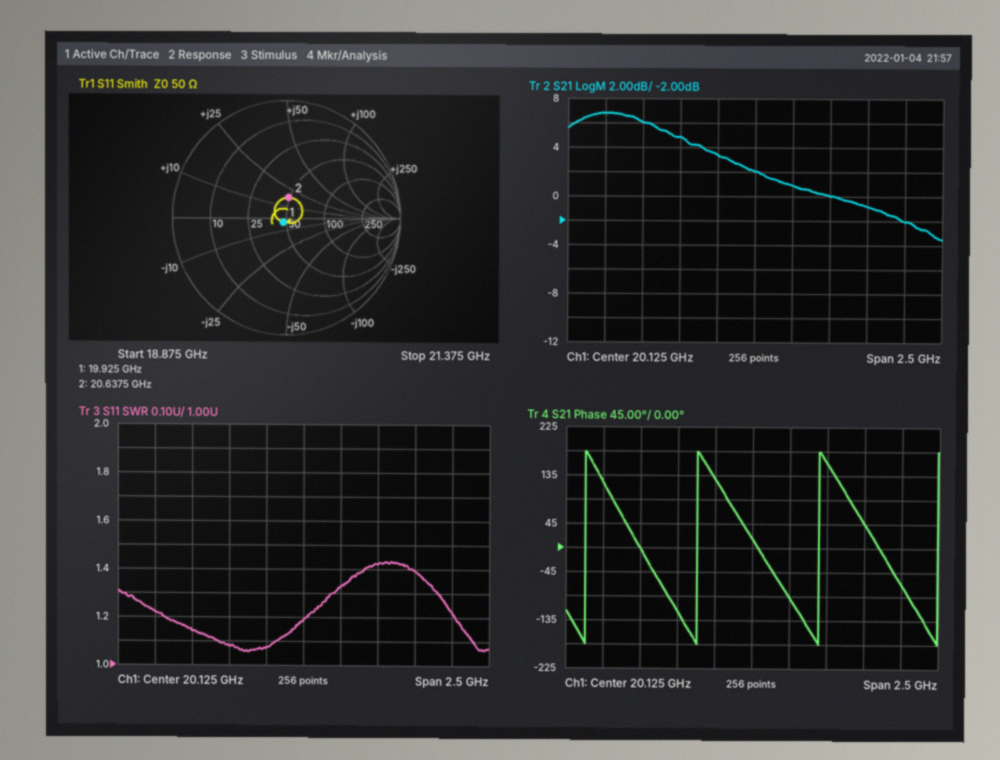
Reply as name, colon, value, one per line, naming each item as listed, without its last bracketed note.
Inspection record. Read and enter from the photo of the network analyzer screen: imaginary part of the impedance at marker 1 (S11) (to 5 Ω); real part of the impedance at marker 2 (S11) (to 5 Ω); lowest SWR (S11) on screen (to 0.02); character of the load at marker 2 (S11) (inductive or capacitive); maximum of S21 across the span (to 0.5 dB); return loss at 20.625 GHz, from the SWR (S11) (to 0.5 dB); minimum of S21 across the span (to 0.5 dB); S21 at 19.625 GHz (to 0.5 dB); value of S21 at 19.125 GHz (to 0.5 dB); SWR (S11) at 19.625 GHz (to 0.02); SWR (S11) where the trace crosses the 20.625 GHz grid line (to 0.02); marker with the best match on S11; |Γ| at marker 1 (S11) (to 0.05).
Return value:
imaginary part of the impedance at marker 1 (S11): -5 Ω
real part of the impedance at marker 2 (S11): 50 Ω
lowest SWR (S11) on screen: 1.06
character of the load at marker 2 (S11): inductive
maximum of S21 across the span: 7.0 dB
return loss at 20.625 GHz, from the SWR (S11): 15.0 dB
minimum of S21 across the span: -3.5 dB
S21 at 19.625 GHz: 5.0 dB
value of S21 at 19.125 GHz: 7.0 dB
SWR (S11) at 19.625 GHz: 1.08
SWR (S11) where the trace crosses the 20.625 GHz grid line: 1.42
marker with the best match on S11: marker 1
|Γ| at marker 1 (S11): 0.05
